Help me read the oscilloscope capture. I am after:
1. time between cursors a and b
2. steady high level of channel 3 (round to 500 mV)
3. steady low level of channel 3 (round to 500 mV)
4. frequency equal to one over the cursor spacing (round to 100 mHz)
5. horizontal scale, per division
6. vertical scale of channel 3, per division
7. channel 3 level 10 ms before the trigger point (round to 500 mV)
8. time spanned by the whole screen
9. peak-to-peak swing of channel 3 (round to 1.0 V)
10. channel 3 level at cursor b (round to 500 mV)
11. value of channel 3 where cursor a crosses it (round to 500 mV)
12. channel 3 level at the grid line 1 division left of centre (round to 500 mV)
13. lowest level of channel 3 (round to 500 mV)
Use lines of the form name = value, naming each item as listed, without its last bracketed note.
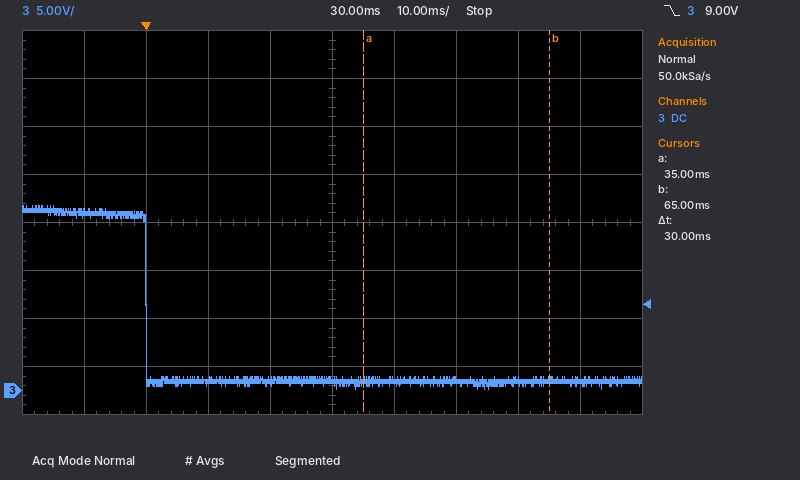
time between cursors a and b = 30 ms
steady high level of channel 3 = 18.5 V
steady low level of channel 3 = 1.0 V
frequency equal to one over the cursor spacing = 33.3 Hz
horizontal scale, per division = 10 ms
vertical scale of channel 3, per division = 5 V
channel 3 level 10 ms before the trigger point = 18.5 V
time spanned by the whole screen = 100 ms
peak-to-peak swing of channel 3 = 19.0 V
channel 3 level at cursor b = 1.0 V
value of channel 3 where cursor a crosses it = 1.0 V
channel 3 level at the grid line 1 division left of centre = 1.0 V
lowest level of channel 3 = 0.0 V
